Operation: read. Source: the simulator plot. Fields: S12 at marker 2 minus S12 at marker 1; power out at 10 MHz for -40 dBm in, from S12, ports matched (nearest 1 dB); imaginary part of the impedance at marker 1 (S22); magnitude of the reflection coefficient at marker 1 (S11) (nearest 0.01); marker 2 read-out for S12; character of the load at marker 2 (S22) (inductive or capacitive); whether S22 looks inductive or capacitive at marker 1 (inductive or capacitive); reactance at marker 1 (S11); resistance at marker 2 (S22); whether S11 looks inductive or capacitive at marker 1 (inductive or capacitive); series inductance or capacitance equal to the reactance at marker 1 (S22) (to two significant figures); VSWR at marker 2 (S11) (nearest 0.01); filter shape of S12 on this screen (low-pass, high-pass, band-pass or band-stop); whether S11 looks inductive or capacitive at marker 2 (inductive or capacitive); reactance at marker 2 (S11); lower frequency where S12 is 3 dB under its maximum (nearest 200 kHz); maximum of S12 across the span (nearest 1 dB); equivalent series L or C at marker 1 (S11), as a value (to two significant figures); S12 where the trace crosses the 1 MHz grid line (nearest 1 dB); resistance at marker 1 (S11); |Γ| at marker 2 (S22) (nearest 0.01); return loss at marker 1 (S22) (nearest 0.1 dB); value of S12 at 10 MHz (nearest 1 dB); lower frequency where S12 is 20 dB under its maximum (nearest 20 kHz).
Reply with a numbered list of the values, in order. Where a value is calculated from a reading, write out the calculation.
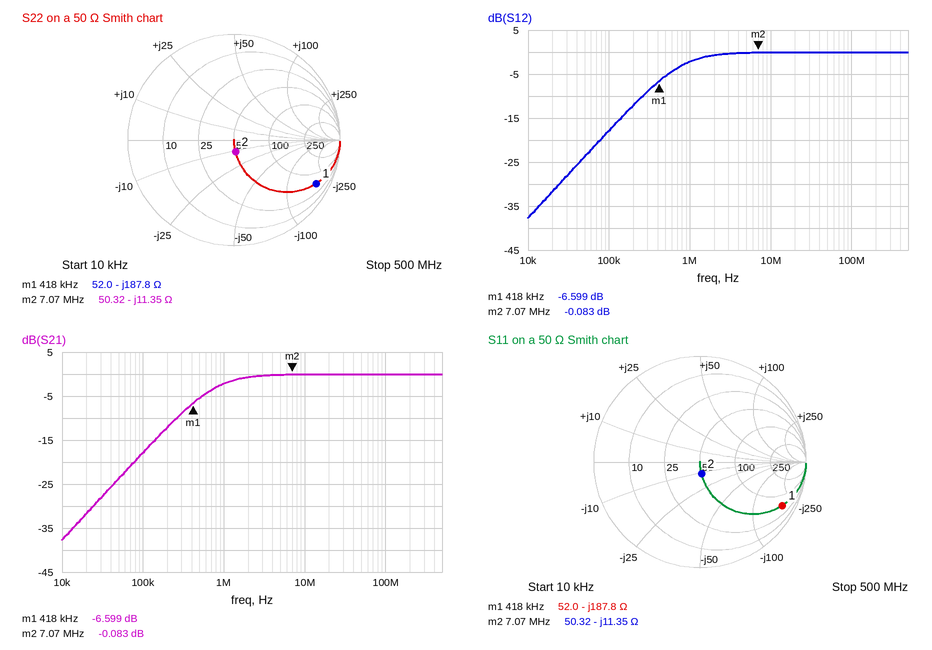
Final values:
1. -0.083 − (-6.599) = 6.516 dB
2. -40 dBm + (0 dB) = -40 dBm
3. -187.8 Ω
4. 0.88
5. -0.083 dB
6. capacitive
7. capacitive
8. -187.8 Ω
9. 50.32 Ω
10. capacitive
11. C = 1/(2π × 418 kHz × 187.8 Ω) ≈ 2.0 nF
12. 1.25
13. high-pass
14. capacitive
15. -11.35 Ω
16. 800 kHz
17. 0 dB
18. C = 1/(2π × 418 kHz × 187.8 Ω) ≈ 2.0 nF
19. -2 dB
20. 52.0 Ω
21. 0.11
22. 1.1 dB
23. 0 dB
24. 80 kHz
